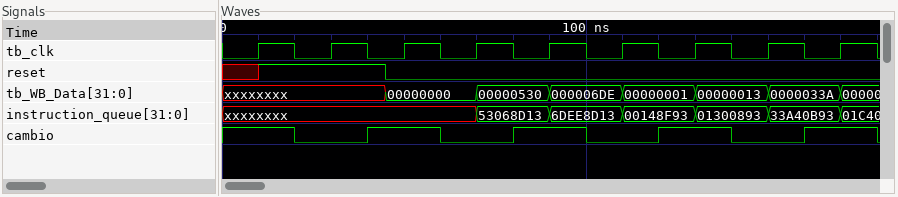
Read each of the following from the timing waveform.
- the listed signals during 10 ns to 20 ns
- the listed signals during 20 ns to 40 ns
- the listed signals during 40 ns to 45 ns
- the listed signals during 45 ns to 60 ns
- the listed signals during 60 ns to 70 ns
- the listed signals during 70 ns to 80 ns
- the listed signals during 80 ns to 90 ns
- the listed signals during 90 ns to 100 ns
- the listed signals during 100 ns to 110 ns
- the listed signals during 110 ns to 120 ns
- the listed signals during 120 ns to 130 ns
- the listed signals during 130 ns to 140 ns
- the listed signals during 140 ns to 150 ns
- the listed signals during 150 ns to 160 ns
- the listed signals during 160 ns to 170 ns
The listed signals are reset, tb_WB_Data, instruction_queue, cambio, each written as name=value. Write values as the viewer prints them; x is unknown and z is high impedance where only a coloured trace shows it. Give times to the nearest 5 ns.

reset=1, tb_WB_Data=xxxxxxxx, instruction_queue=xxxxxxxx, cambio=1
reset=1, tb_WB_Data=xxxxxxxx, instruction_queue=xxxxxxxx, cambio=0
reset=1, tb_WB_Data=xxxxxxxx, instruction_queue=xxxxxxxx, cambio=1
reset=0, tb_WB_Data=00000000, instruction_queue=xxxxxxxx, cambio=1
reset=0, tb_WB_Data=00000000, instruction_queue=xxxxxxxx, cambio=0
reset=0, tb_WB_Data=00000530, instruction_queue=53068D13, cambio=0
reset=0, tb_WB_Data=00000530, instruction_queue=53068D13, cambio=1
reset=0, tb_WB_Data=000006DE, instruction_queue=6DEE8D13, cambio=1
reset=0, tb_WB_Data=000006DE, instruction_queue=6DEE8D13, cambio=0
reset=0, tb_WB_Data=00000001, instruction_queue=00148F93, cambio=0
reset=0, tb_WB_Data=00000001, instruction_queue=00148F93, cambio=1
reset=0, tb_WB_Data=00000013, instruction_queue=01300893, cambio=1
reset=0, tb_WB_Data=00000013, instruction_queue=01300893, cambio=0
reset=0, tb_WB_Data=0000033A, instruction_queue=33A40B93, cambio=0
reset=0, tb_WB_Data=0000033A, instruction_queue=33A40B93, cambio=1
